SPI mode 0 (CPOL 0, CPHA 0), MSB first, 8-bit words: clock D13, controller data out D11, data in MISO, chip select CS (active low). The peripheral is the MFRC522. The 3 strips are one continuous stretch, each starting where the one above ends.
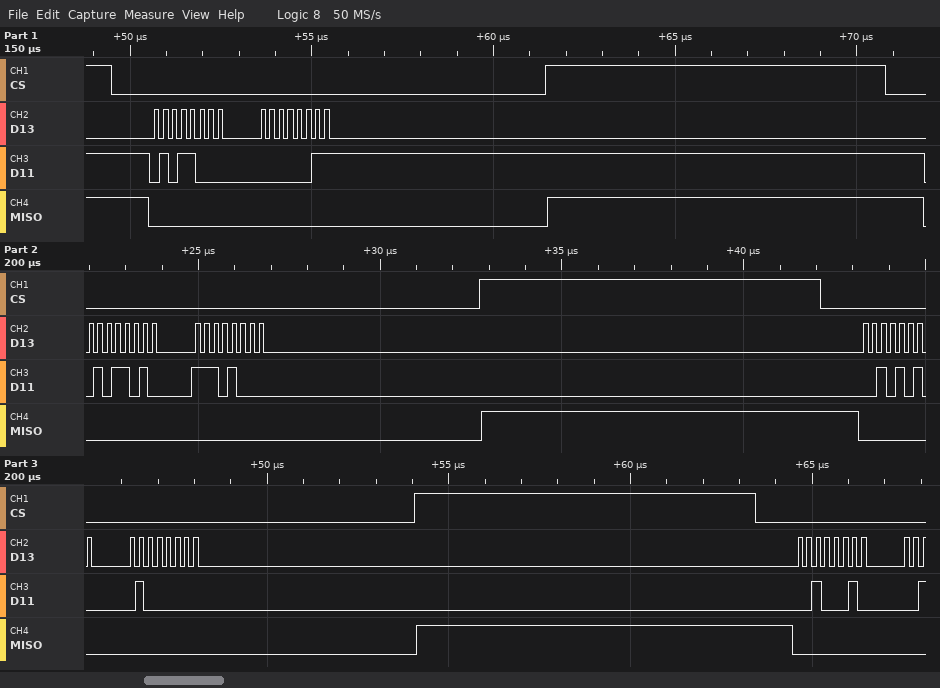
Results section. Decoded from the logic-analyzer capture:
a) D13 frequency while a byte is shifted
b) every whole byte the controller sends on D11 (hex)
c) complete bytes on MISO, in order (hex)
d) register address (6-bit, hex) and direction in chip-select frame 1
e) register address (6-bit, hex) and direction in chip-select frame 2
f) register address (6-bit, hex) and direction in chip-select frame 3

4 MHz
58 03 5A E8 2A 40 22
00 00 00 00 00 00 00
0x2C write
0x2D write
0x15 write
